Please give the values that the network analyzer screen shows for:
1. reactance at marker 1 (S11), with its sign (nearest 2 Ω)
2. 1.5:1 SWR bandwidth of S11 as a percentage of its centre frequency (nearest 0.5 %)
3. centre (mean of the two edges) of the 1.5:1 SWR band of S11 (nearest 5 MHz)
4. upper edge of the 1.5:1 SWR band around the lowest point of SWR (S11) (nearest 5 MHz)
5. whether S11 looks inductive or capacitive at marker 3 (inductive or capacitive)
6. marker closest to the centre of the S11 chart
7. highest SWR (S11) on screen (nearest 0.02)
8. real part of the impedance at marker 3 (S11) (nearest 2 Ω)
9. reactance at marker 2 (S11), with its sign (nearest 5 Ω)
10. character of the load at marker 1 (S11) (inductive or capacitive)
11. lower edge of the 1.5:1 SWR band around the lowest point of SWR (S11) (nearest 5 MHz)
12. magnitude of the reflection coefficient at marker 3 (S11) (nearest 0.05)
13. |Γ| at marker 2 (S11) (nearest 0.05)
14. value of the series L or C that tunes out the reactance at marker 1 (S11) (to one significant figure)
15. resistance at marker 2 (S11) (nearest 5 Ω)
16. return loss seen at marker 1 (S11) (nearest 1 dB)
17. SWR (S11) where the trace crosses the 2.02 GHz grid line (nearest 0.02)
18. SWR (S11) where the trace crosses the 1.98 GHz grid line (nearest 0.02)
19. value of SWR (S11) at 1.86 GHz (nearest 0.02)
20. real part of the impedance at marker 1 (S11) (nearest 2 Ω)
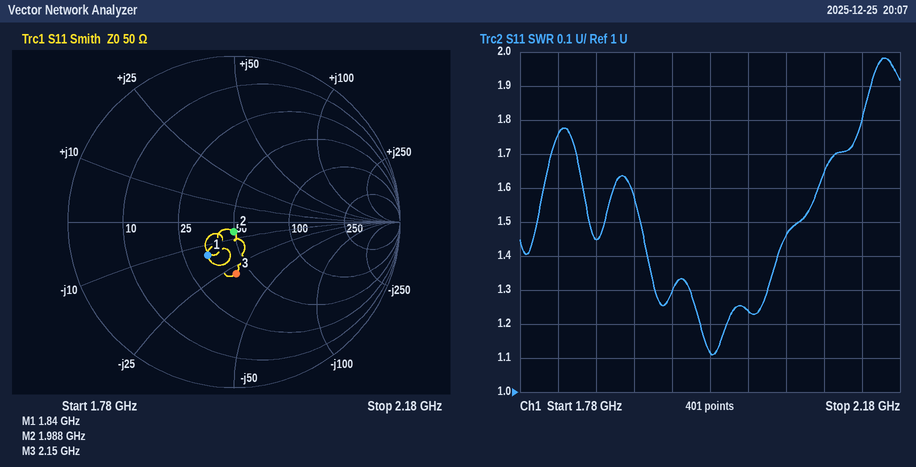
-14 Ω
8.5 %
1.990 GHz
2.075 GHz
capacitive
marker 2
1.98
42 Ω
-5 Ω
capacitive
1.905 GHz
0.30
0.05
1 nH
50 Ω
12 dB
1.24
1.12
1.44
34 Ω
